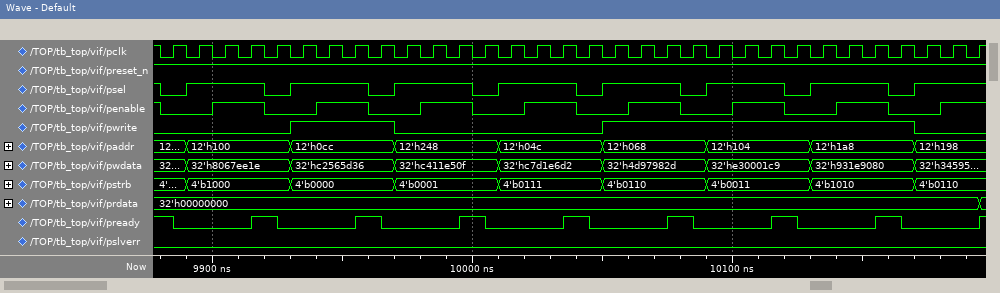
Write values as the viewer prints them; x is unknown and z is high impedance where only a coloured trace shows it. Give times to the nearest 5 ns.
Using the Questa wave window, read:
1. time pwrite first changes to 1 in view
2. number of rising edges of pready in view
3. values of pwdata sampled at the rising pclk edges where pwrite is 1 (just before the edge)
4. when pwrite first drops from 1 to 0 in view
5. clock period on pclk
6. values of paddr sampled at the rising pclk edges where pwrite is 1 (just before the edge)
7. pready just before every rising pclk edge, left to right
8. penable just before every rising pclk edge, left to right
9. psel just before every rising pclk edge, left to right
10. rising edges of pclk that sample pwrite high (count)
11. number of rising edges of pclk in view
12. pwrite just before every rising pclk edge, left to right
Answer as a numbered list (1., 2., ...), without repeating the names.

1. 9930 ns
2. 8
3. 32'hc2565d36, 32'hc2565d36, 32'hc2565d36, 32'hc2565d36, 32'h4d97982d, 32'h4d97982d, 32'h4d97982d, 32'h4d97982d, 32'he30001c9, 32'he30001c9, 32'he30001c9, 32'he30001c9, 32'h931e9080, 32'h931e9080, 32'h931e9080, 32'h931e9080
4. 9970 ns
5. 10 ns
6. 12'h0cc, 12'h0cc, 12'h0cc, 12'h0cc, 12'h068, 12'h068, 12'h068, 12'h068, 12'h104, 12'h104, 12'h104, 12'h104, 12'h1a8, 12'h1a8, 12'h1a8, 12'h1a8
7. 1 0 0 0 1 0 0 0 1 0 0 0 1 0 0 0 1 0 0 0 1 0 0 0 1 0 0 0 1 0 0 0
8. 0 0 1 1 0 0 1 1 0 0 1 1 0 0 1 1 0 0 1 1 0 0 1 1 0 0 1 1 0 0 1 1
9. 0 1 1 1 0 1 1 1 0 1 1 1 0 1 1 1 0 1 1 1 0 1 1 1 0 1 1 1 0 1 1 1
10. 16
11. 32
12. 0 0 0 0 0 1 1 1 1 0 0 0 0 0 0 0 0 1 1 1 1 1 1 1 1 1 1 1 1 0 0 0
